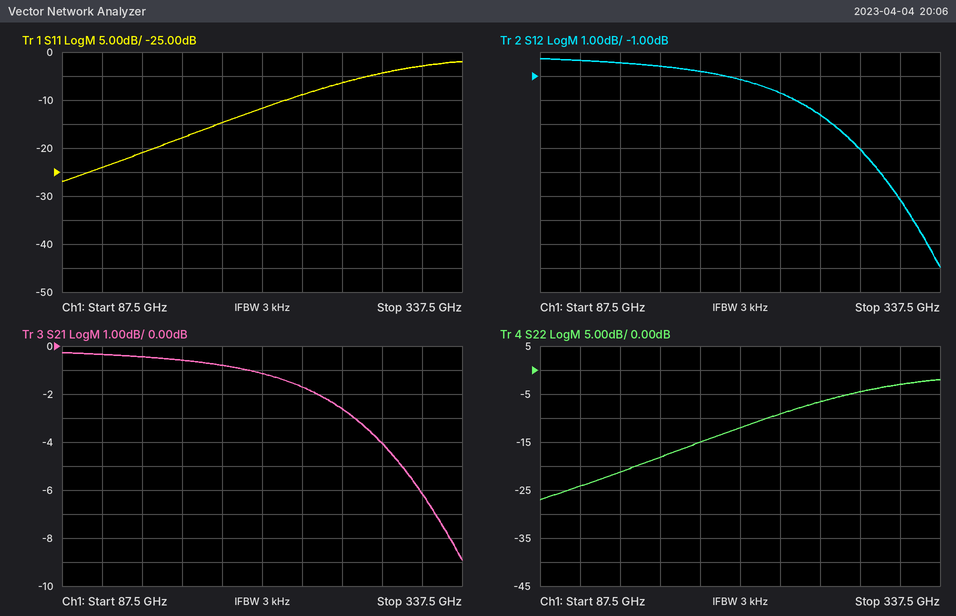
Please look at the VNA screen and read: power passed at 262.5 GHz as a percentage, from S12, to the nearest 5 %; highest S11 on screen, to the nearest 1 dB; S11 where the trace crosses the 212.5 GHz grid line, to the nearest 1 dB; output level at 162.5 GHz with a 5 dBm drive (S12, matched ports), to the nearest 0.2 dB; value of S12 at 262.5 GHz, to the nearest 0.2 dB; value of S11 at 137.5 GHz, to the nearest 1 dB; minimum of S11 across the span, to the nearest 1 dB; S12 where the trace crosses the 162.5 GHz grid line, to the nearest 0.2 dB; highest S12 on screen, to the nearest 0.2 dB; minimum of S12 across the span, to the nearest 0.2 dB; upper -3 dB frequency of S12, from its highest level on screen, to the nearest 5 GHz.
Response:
55 %
-2 dB
-12 dB
4.4 dBm
-2.6 dB
-21 dB
-27 dB
-0.6 dB
-0.2 dB
-9.0 dB
275 GHz
